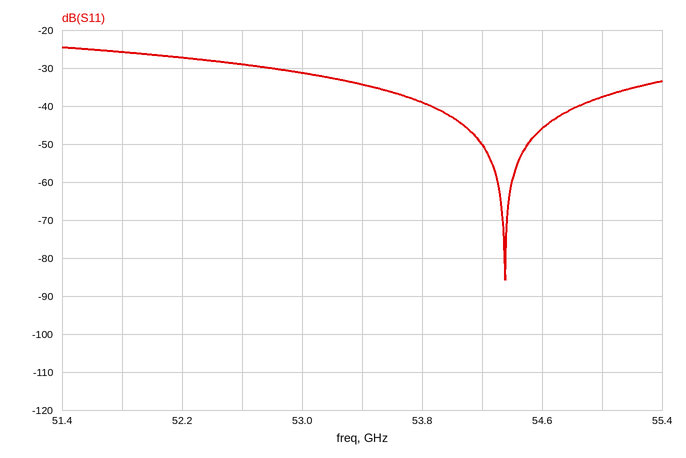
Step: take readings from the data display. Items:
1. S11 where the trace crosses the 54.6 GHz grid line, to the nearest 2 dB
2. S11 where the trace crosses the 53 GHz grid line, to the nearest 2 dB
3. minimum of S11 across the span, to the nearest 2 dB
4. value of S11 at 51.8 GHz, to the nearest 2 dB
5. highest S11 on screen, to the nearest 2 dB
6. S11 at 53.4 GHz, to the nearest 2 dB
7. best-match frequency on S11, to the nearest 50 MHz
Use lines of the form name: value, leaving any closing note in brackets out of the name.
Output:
S11 where the trace crosses the 54.6 GHz grid line, to the nearest 2 dB: -46 dB
S11 where the trace crosses the 53 GHz grid line, to the nearest 2 dB: -32 dB
minimum of S11 across the span, to the nearest 2 dB: -86 dB
value of S11 at 51.8 GHz, to the nearest 2 dB: -26 dB
highest S11 on screen, to the nearest 2 dB: -24 dB
S11 at 53.4 GHz, to the nearest 2 dB: -34 dB
best-match frequency on S11, to the nearest 50 MHz: 54.35 GHz
